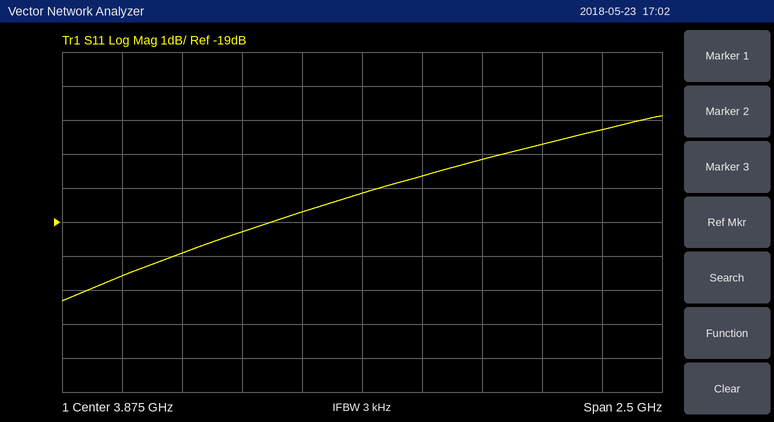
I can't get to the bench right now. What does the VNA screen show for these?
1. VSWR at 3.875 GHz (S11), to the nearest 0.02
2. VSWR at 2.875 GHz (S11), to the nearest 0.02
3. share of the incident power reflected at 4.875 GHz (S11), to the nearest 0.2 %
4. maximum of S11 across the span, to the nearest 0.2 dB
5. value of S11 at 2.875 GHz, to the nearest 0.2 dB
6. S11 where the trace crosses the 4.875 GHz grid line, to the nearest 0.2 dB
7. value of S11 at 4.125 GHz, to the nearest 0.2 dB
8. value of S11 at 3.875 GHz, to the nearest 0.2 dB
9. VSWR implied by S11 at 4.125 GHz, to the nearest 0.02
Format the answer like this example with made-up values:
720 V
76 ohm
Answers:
1.28
1.20
2.4 %
-15.8 dB
-20.6 dB
-16.2 dB
-17.6 dB
-18.2 dB
1.30
